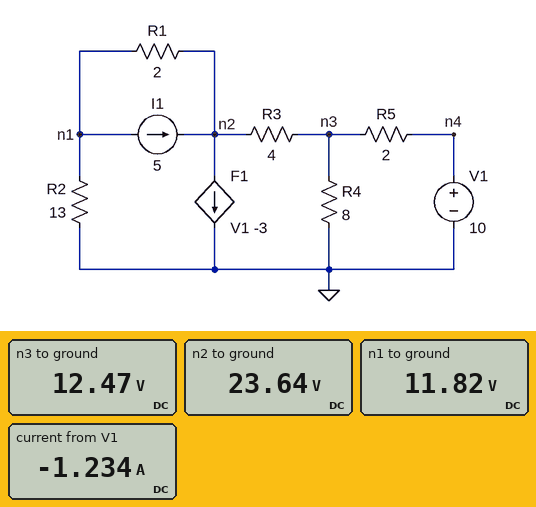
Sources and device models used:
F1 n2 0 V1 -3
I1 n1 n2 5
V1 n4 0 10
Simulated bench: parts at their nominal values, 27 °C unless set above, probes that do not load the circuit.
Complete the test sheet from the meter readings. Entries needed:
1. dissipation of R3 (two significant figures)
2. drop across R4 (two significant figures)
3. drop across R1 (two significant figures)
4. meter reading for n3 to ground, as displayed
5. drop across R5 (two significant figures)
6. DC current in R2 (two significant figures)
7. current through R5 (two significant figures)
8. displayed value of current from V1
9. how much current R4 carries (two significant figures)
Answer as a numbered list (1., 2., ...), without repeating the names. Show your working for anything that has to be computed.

1. (23.64 V - 12.47 V)^2 / 4 Ω = 31 W
2. 12.47 V = 12 V
3. 23.64 V - 11.82 V = 12 V
4. 12.47 V
5. 12.47 V - 10 V = 2.5 V
6. (11.82 V) / 13 Ω = 910 mA
7. (12.47 V - 10 V) / 2 Ω = 1.2 A
8. -1.234 A
9. (12.47 V) / 8 Ω = 1.6 A
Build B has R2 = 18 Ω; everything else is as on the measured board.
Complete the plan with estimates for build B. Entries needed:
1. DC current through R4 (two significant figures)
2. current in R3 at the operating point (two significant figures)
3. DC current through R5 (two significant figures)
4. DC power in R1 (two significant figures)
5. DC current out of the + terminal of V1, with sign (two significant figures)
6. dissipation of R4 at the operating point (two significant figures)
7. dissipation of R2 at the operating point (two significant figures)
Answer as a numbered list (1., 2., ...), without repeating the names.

1. 1.5 A
2. 2.6 A
3. 1.1 A
4. 63 W
5. -1.1 A
6. 18 W
7. 7.0 W
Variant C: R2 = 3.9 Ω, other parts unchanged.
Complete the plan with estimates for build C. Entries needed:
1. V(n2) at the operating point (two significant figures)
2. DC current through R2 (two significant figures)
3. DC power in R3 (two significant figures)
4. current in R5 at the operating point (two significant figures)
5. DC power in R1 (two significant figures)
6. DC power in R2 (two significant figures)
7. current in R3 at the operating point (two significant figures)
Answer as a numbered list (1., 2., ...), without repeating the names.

1. 41 V
2. 5.3 A
3. 140 W
4. 3.7 A
5. 210 W
6. 110 W
7. 5.9 A
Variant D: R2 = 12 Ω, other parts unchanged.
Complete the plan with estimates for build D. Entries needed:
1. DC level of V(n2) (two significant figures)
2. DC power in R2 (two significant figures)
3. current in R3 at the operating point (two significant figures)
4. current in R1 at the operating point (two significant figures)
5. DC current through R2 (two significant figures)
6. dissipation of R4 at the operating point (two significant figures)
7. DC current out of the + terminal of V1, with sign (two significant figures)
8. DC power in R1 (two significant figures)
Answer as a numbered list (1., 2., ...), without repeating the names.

1. 24 V
2. 12 W
3. 2.9 A
4. 6.0 A
5. 1.0 A
6. 20 W
7. -1.3 A
8. 72 W
